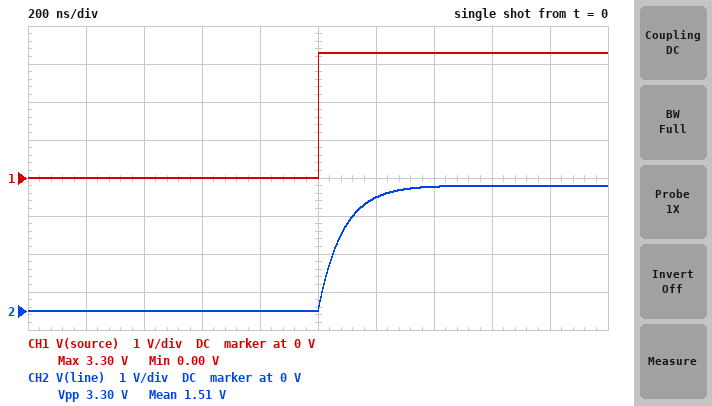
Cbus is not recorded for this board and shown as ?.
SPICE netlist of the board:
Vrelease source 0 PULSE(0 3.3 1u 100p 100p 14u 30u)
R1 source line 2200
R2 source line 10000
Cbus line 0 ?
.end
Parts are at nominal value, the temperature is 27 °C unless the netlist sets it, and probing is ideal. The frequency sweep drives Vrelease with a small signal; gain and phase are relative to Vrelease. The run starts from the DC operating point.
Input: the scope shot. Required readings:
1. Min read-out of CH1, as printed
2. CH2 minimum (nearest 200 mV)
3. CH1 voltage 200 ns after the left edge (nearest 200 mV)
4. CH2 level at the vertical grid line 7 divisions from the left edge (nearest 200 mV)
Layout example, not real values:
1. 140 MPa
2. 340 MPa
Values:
1. 0.00 V
2. 0 V
3. 0 V
4. 3.2 V
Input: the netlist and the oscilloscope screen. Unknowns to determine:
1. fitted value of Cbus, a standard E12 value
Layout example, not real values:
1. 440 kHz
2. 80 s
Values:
1. 47 pF
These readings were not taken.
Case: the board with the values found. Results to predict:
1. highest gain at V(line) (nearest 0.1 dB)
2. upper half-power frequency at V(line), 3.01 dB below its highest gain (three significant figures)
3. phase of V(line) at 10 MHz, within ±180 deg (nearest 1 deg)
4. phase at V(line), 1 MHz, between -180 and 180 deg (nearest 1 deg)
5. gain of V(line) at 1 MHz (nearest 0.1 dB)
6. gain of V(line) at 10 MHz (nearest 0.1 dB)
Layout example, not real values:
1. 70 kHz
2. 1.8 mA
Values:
1. 0 dB
2. 1.88 MHz
3. -79 deg
4. -28 deg
5. -1.1 dB
6. -14.7 dB
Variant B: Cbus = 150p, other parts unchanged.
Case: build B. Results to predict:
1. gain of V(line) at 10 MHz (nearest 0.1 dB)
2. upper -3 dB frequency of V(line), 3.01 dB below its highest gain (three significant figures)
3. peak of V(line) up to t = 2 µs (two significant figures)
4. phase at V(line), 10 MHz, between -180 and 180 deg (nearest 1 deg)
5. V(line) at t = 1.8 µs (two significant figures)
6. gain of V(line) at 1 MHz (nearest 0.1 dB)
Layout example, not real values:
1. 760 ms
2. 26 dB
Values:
1. -24.6 dB
2. 588 kHz
3. 3.2 V
4. -87 deg
5. 3.1 V
6. -5.9 dB
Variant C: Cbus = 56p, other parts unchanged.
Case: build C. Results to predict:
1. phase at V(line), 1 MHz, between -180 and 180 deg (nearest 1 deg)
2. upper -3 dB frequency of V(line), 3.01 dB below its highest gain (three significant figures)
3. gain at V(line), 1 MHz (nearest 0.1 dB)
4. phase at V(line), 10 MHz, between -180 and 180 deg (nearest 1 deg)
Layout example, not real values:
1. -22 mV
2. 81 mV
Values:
1. -32 deg
2. 1.58 MHz
3. -1.5 dB
4. -81 deg
